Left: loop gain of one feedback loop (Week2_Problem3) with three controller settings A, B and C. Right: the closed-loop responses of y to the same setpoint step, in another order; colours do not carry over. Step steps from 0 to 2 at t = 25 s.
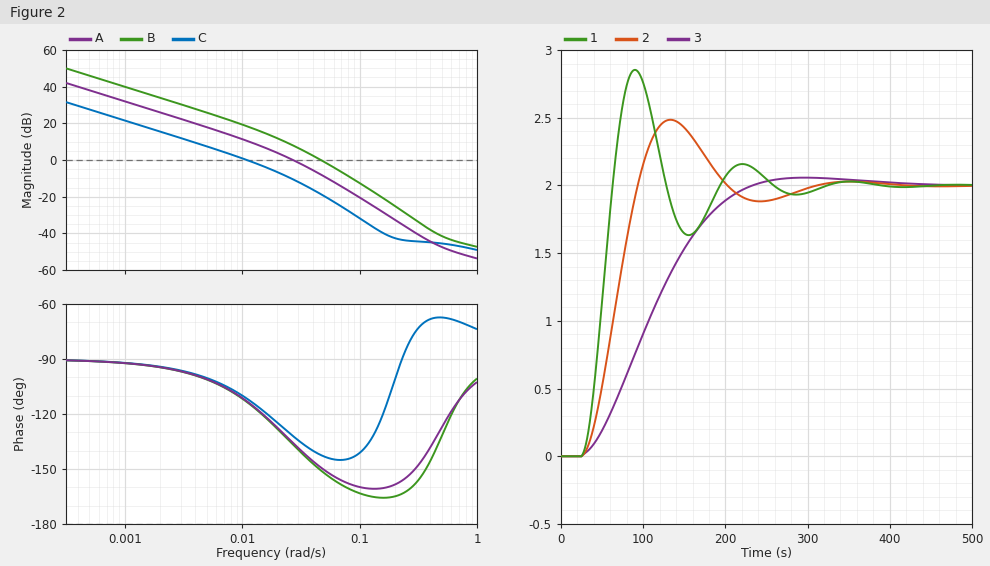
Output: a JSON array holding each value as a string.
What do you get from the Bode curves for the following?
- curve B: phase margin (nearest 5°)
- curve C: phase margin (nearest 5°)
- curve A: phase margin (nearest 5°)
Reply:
["30°", "70°", "45°"]
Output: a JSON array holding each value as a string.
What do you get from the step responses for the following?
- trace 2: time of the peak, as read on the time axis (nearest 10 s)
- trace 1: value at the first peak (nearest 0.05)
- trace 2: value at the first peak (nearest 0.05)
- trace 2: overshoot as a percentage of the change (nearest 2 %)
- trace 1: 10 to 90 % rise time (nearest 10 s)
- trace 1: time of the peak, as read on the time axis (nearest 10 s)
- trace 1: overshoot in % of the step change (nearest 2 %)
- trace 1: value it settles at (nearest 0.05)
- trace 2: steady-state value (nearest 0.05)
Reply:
["130 s", "2.85", "2.50", "24 %", "30 s", "90 s", "42 %", "2.00", "2.00"]
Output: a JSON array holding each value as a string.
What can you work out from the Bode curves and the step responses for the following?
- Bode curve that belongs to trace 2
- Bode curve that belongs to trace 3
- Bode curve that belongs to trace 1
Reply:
["A", "C", "B"]
